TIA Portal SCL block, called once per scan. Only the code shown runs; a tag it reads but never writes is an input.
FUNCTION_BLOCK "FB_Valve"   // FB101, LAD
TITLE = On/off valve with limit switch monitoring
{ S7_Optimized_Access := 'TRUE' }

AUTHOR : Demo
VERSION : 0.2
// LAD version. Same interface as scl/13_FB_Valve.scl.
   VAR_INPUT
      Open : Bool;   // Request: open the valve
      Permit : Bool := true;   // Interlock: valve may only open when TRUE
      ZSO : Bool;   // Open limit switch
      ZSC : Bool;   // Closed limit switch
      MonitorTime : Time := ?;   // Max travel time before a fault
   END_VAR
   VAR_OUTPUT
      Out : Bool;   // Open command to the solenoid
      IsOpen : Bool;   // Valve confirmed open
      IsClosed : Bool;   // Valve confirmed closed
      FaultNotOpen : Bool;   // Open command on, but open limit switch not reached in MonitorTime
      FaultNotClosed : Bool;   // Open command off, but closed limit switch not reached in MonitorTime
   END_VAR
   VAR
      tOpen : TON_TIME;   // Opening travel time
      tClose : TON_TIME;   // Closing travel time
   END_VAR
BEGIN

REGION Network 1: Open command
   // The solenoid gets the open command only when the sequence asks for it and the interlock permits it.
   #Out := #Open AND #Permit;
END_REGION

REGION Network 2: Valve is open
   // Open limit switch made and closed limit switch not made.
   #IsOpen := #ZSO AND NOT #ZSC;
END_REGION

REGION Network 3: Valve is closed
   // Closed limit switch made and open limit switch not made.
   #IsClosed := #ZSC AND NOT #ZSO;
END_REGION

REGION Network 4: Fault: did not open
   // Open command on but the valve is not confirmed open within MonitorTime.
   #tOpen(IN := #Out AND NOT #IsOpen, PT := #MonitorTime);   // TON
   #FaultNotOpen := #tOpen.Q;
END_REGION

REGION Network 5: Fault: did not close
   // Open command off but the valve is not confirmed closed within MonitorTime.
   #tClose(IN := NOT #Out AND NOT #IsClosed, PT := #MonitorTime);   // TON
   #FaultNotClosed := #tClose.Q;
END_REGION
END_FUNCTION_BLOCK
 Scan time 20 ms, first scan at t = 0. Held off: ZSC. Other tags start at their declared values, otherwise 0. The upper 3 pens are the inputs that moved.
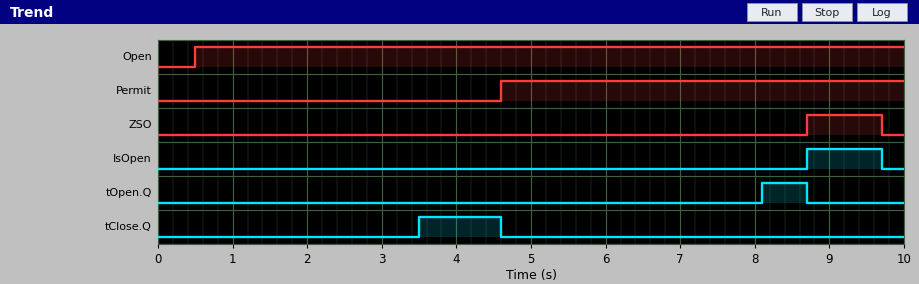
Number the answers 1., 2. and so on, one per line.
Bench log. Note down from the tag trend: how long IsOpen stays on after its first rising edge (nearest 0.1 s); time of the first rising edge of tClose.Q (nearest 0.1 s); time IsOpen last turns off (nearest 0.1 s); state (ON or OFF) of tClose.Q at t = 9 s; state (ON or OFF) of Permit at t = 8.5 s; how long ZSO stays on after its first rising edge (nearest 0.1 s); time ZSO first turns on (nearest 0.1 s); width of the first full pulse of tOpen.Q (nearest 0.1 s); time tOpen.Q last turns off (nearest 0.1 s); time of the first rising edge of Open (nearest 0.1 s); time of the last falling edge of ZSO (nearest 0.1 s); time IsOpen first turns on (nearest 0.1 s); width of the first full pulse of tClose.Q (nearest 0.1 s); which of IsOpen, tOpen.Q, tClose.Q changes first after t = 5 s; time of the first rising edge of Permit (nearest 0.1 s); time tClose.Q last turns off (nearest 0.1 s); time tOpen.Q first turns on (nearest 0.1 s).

1. 1.0 s
2. 3.5 s
3. 9.7 s
4. OFF
5. ON
6. 1.0 s
7. 8.7 s
8. 0.6 s
9. 8.7 s
10. 0.5 s
11. 9.7 s
12. 8.7 s
13. 1.1 s
14. tOpen.Q
15. 4.6 s
16. 4.6 s
17. 8.1 s
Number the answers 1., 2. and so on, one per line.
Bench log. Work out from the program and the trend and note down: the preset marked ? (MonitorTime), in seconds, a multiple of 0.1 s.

1. 3.5 s
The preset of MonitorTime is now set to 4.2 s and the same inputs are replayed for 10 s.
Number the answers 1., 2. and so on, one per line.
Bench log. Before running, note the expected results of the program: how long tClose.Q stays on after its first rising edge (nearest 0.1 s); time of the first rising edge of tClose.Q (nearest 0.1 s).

1. 0.4 s
2. 4.2 s
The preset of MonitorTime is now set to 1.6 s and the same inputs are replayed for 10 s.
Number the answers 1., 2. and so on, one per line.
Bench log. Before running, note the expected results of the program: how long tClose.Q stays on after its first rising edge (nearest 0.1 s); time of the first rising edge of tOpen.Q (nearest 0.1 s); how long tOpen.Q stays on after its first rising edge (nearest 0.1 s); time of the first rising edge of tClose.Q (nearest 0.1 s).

1. 3.0 s
2. 6.2 s
3. 2.5 s
4. 1.6 s
